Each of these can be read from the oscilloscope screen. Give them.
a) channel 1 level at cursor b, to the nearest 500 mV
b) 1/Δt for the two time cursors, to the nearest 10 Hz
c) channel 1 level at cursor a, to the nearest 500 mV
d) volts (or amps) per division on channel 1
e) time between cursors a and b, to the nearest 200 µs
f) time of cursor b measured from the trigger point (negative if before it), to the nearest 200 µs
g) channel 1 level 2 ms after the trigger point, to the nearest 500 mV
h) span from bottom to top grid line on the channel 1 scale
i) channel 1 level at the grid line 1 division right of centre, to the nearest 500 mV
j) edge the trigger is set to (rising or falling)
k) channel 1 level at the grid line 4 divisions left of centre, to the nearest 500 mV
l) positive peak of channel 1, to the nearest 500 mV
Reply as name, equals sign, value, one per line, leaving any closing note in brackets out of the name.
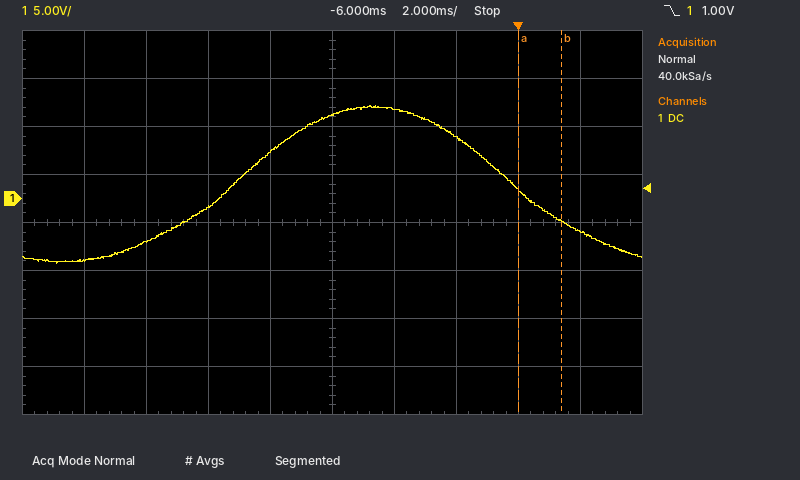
channel 1 level at cursor b, to the nearest 500 mV = -2.5 V
1/Δt for the two time cursors, to the nearest 10 Hz = 710 Hz
channel 1 level at cursor a, to the nearest 500 mV = 1.0 V
volts (or amps) per division on channel 1 = 5 V
time between cursors a and b, to the nearest 200 µs = 1.4 ms
time of cursor b measured from the trigger point (negative if before it), to the nearest 200 µs = +1.4 ms
channel 1 level 2 ms after the trigger point, to the nearest 500 mV = -3.5 V
span from bottom to top grid line on the channel 1 scale = 40 V
channel 1 level at the grid line 1 division right of centre, to the nearest 500 mV = 9.5 V
edge the trigger is set to = falling
channel 1 level at the grid line 4 divisions left of centre, to the nearest 500 mV = -6.5 V
positive peak of channel 1, to the nearest 500 mV = 9.5 V
